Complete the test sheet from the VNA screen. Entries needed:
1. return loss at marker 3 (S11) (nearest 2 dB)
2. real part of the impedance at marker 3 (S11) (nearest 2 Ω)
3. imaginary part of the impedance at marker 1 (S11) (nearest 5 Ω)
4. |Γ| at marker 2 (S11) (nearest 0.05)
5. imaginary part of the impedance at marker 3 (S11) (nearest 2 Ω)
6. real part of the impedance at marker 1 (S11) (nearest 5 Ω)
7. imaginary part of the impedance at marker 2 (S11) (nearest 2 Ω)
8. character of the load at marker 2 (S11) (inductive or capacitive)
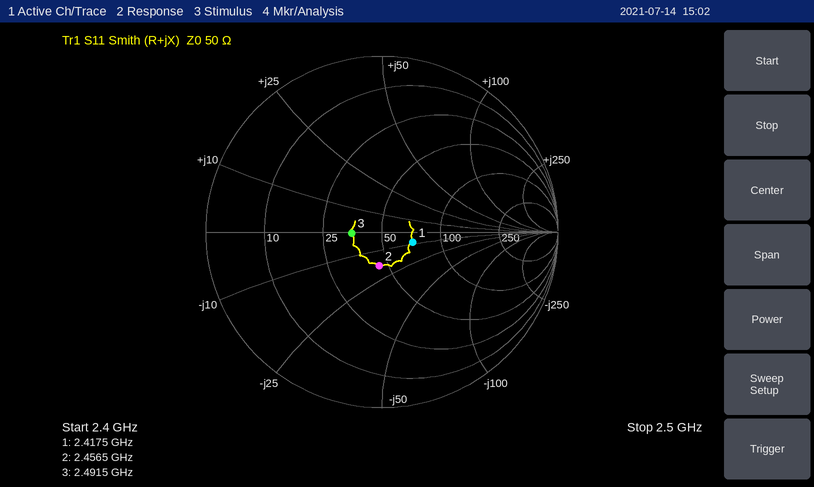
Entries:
16 dB
36 Ω
-10 Ω
0.20
0 Ω
70 Ω
-18 Ω
capacitive
